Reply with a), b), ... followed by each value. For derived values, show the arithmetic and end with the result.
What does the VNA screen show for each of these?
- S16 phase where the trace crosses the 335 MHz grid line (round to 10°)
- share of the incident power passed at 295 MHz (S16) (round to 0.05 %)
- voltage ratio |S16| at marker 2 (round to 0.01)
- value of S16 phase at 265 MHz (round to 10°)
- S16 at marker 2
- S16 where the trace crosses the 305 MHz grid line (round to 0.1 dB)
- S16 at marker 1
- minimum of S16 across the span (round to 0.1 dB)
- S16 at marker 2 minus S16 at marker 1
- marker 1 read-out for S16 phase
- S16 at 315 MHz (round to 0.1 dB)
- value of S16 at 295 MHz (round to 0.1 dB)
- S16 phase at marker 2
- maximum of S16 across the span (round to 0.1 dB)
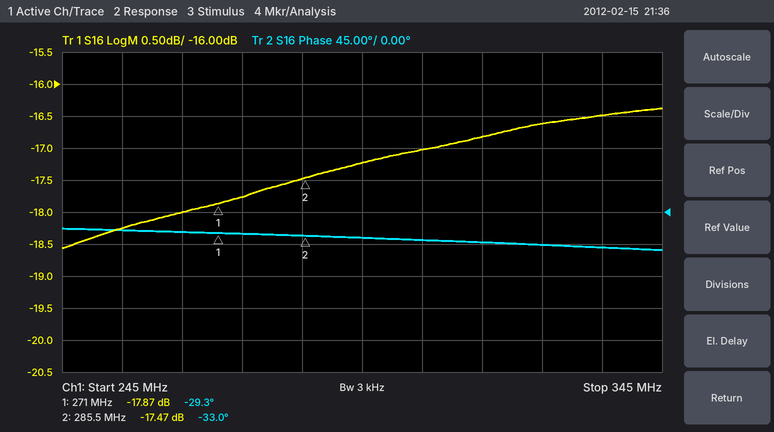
a) -50°
b) 10^(-17.2/10) ≈ 1.91 %, so 1.90 % to the nearest 0.05 %
c) 10^(-17.47/20) ≈ 0.13
d) -30°
e) -17.47 dB
f) -17.0 dB
g) -17.87 dB
h) -18.6 dB
i) -17.47 − (-17.87) = 0.40 dB
j) -29.3°
k) -16.8 dB
l) -17.2 dB
m) -33.0°
n) -16.4 dB
